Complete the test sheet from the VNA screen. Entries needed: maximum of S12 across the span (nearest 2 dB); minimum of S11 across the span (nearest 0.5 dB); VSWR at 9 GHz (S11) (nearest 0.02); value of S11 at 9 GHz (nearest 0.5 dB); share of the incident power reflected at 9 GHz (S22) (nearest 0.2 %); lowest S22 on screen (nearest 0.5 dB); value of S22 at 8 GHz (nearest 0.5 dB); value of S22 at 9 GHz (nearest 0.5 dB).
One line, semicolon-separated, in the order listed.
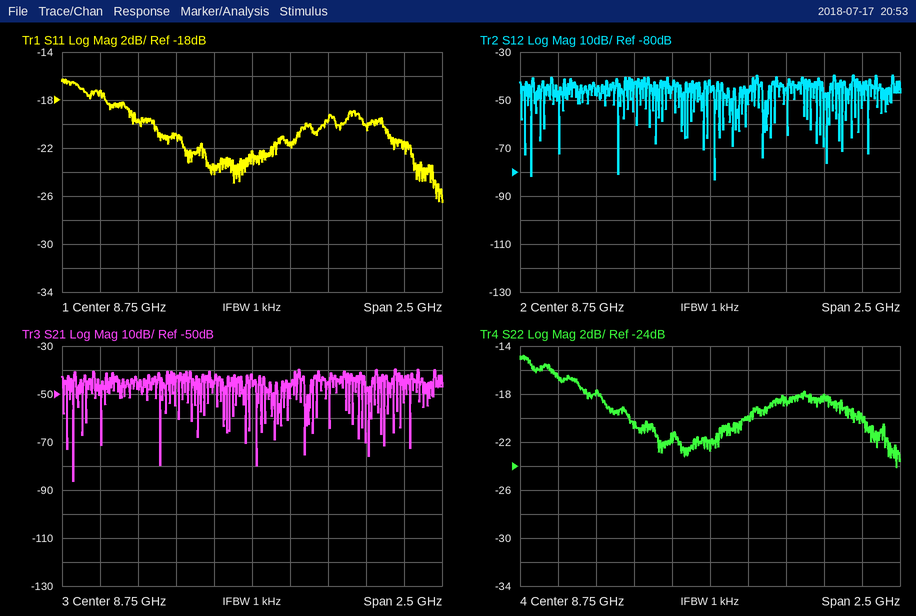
-40 dB; -26.5 dB; 1.18; -21.5 dB; 1.0 %; -24.0 dB; -18.0 dB; -20.0 dB
